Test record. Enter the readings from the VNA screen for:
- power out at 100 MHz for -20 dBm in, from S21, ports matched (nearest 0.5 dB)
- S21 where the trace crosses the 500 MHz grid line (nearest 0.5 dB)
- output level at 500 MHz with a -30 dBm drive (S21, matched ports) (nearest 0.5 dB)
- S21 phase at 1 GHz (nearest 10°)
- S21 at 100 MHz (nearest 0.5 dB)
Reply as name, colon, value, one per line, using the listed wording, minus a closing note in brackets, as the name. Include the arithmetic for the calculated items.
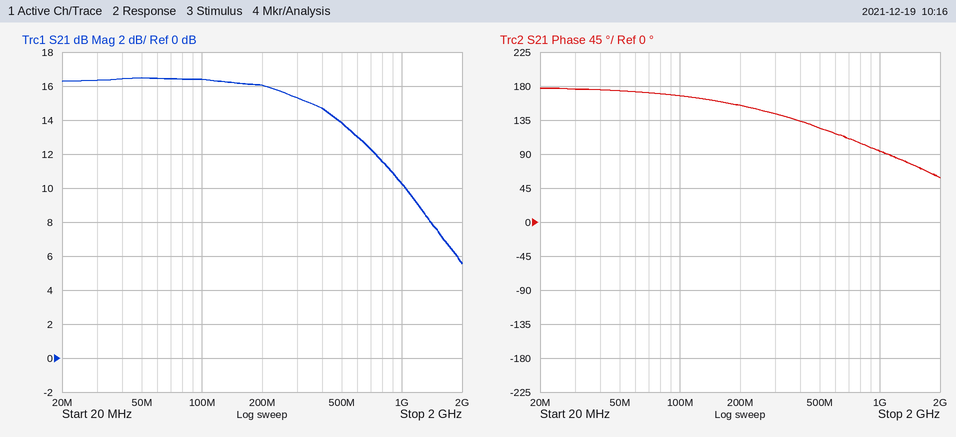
power out at 100 MHz for -20 dBm in, from S21, ports matched: -20 dBm + (16.5 dB) = -3.5 dBm
S21 where the trace crosses the 500 MHz grid line: 14.0 dB
output level at 500 MHz with a -30 dBm drive (S21, matched ports): -30 dBm + (14.0 dB) = -16.0 dBm
S21 phase at 1 GHz: 90°
S21 at 100 MHz: 16.5 dB
